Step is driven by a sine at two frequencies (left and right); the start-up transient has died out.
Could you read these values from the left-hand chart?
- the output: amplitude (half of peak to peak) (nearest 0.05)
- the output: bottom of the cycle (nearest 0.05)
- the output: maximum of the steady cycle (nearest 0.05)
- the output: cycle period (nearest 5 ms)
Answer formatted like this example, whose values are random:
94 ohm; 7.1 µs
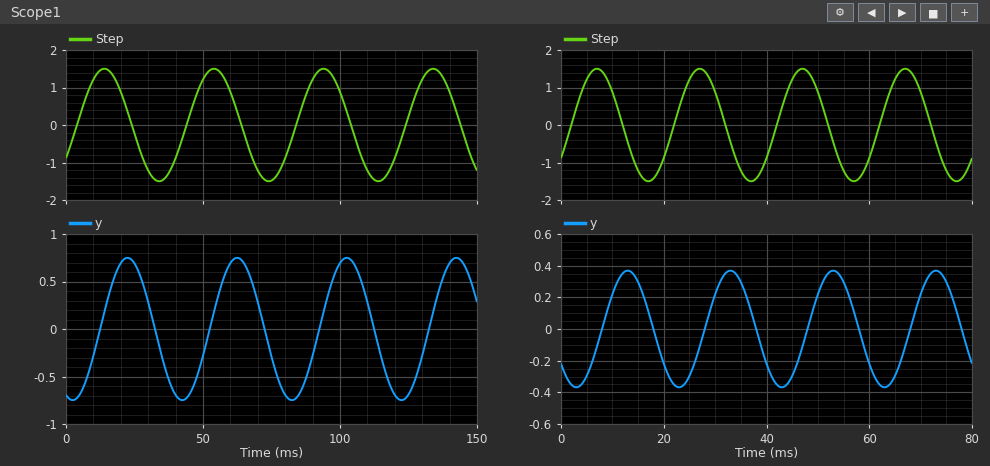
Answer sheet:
0.75; -0.75; 0.75; 40 ms
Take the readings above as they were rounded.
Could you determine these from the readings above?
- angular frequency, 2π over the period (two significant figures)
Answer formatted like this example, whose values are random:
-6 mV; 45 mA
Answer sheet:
0.16 rad/ms
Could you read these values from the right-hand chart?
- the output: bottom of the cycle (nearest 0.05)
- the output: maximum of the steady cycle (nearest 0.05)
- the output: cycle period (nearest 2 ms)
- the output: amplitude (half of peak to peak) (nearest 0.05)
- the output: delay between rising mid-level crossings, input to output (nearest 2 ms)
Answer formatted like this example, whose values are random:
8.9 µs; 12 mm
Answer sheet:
-0.35; 0.35; 20 ms; 0.35; 6 ms
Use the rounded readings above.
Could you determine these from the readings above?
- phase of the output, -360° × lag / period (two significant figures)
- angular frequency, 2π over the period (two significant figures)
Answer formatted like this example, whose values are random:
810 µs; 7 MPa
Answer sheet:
-110°; 0.31 rad/ms
